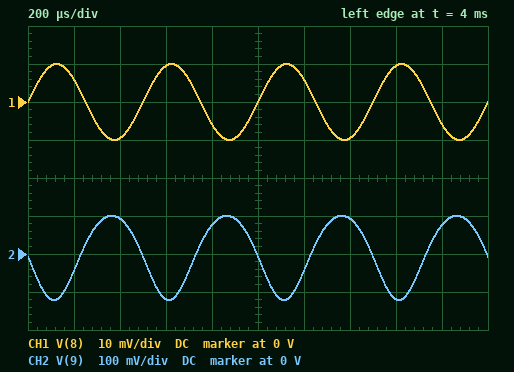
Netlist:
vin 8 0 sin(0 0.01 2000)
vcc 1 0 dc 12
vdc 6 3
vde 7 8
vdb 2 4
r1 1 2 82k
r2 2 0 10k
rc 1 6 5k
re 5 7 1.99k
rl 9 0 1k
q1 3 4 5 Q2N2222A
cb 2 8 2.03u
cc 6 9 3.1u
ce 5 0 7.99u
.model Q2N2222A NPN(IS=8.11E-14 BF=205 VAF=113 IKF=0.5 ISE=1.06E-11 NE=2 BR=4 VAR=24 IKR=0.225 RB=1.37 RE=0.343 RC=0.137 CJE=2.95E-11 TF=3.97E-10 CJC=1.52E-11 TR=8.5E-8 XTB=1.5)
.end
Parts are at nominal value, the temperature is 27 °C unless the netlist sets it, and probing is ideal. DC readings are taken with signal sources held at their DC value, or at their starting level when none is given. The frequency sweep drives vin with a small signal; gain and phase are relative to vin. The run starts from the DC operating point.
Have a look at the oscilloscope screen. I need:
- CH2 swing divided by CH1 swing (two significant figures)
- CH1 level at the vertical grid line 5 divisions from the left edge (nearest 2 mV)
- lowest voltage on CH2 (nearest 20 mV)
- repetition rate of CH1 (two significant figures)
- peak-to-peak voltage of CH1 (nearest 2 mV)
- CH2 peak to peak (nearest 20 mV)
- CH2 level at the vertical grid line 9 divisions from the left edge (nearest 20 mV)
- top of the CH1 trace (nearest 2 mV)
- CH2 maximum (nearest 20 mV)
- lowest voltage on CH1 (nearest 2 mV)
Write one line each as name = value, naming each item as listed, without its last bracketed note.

CH2 swing divided by CH1 swing = 11
CH1 level at the vertical grid line 5 divisions from the left edge = 0 V
lowest voltage on CH2 = -120 mV
repetition rate of CH1 = 2.0 kHz
peak-to-peak voltage of CH1 = 20 mV
CH2 peak to peak = 220 mV
CH2 level at the vertical grid line 9 divisions from the left edge = 80 mV
top of the CH1 trace = 10 mV
CH2 maximum = 100 mV
lowest voltage on CH1 = -10 mV
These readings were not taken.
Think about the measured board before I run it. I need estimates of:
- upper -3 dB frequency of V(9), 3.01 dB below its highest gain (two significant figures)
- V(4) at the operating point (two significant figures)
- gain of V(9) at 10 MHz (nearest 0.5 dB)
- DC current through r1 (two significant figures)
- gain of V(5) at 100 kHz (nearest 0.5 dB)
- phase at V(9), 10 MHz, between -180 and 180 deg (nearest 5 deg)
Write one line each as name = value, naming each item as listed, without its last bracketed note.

upper -3 dB frequency of V(9), 3.01 dB below its highest gain = 29 MHz
V(4) at the operating point = 1.3 V
gain of V(9) at 10 MHz = 20.5 dB
DC current through r1 = 130 µA
gain of V(5) at 100 kHz = -51.0 dB
phase at V(9), 10 MHz, between -180 and 180 deg = 160 deg
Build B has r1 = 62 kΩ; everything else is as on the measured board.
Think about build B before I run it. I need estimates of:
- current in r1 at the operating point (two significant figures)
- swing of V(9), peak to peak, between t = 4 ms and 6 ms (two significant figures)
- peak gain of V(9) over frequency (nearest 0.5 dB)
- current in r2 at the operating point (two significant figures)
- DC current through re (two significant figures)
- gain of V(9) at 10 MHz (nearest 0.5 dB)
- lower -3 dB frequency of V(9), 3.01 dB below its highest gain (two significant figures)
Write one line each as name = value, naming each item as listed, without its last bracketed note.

current in r1 at the operating point = 170 µA
swing of V(9), peak to peak, between t = 4 ms and 6 ms = 320 mV
peak gain of V(9) over frequency = 24.5 dB
current in r2 at the operating point = 160 µA
DC current through re = 530 µA
gain of V(9) at 10 MHz = 24.0 dB
lower -3 dB frequency of V(9), 3.01 dB below its highest gain = 420 Hz
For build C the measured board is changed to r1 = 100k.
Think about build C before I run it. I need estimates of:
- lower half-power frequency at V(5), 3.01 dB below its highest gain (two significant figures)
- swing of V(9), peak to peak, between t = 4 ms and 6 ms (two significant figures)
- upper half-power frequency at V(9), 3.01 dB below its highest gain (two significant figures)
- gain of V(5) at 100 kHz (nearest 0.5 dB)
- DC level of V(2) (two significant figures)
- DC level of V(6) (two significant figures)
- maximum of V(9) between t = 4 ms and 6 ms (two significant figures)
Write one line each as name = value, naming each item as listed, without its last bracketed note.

lower half-power frequency at V(5), 3.01 dB below its highest gain = 8.0 Hz
swing of V(9), peak to peak, between t = 4 ms and 6 ms = 160 mV
upper half-power frequency at V(9), 3.01 dB below its highest gain = 30 MHz
gain of V(5) at 100 kHz = -53.5 dB
DC level of V(2) = 1.1 V
DC level of V(6) = 11 V
maximum of V(9) between t = 4 ms and 6 ms = 73 mV
